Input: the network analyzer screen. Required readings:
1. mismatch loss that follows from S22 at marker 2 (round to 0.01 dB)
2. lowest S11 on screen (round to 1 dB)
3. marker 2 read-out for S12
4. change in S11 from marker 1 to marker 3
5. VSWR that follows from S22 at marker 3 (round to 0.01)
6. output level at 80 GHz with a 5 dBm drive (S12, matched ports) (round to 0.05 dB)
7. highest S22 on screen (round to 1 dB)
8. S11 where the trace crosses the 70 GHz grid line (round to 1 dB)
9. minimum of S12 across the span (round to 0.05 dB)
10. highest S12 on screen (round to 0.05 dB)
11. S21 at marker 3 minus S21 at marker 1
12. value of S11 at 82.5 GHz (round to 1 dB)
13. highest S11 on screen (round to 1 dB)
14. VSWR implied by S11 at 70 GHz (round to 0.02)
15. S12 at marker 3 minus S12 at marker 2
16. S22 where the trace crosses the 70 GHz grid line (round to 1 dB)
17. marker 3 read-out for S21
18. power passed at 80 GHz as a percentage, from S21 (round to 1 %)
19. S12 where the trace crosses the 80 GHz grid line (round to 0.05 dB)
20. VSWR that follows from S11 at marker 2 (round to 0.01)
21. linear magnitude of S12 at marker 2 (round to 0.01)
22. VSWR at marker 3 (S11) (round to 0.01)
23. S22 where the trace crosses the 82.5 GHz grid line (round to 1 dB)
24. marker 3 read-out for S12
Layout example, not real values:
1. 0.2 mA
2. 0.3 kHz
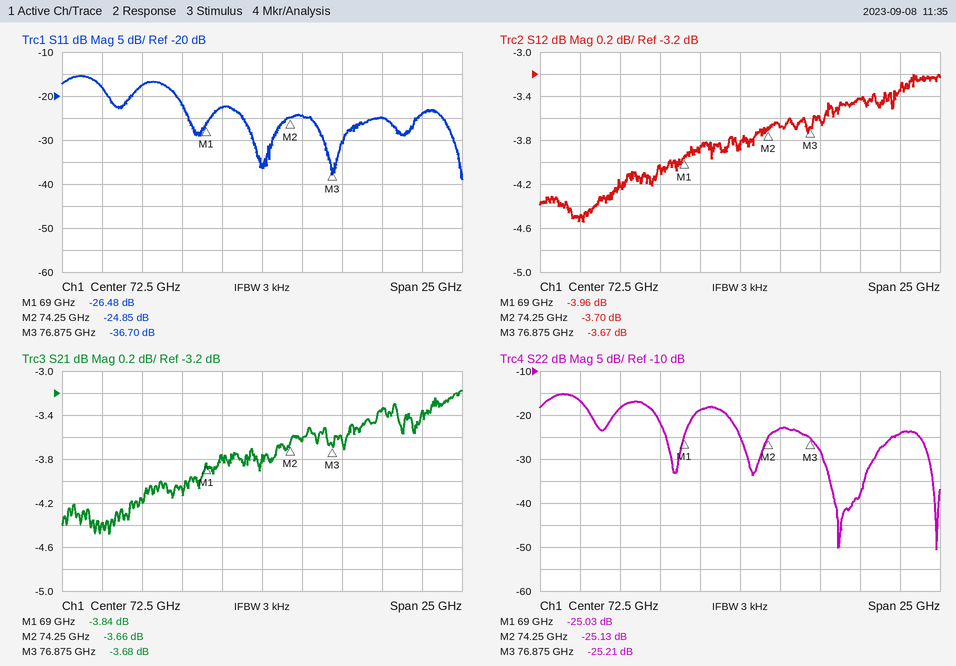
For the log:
1. 0.01 dB
2. -39 dB
3. -3.70 dB
4. -10.22 dB
5. 1.12
6. 1.60 dBm
7. -15 dB
8. -23 dB
9. -4.55 dB
10. -3.20 dB
11. 0.16 dB
12. -24 dB
13. -15 dB
14. 1.16
15. 0.03 dB
16. -19 dB
17. -3.68 dB
18. 46 %
19. -3.40 dB
20. 1.12
21. 0.65
22. 1.03
23. -24 dB
24. -3.67 dB
